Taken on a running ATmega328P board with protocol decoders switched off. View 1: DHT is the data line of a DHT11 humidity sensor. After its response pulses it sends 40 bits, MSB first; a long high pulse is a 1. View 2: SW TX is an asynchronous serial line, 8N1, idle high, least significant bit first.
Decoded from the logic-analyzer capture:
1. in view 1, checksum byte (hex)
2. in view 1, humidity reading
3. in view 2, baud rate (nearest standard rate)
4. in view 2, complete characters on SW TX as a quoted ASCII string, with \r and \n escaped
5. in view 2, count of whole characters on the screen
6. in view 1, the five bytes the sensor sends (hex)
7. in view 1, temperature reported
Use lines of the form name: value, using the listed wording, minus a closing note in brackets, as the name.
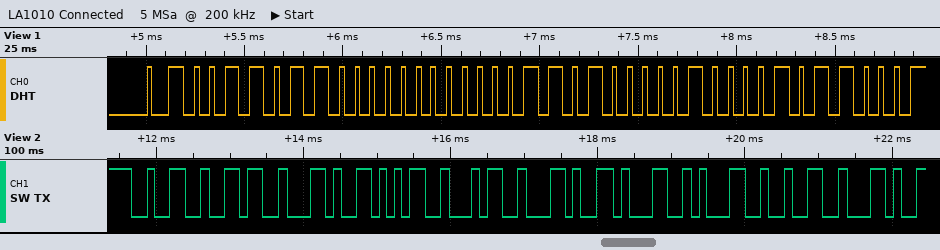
in view 1, checksum byte: 0x58
in view 1, humidity reading: 54 %
in view 2, baud rate: 9600 baud
in view 2, complete characters on SW TX as a quoted ASCII string, with \r and \n escaped: "26,54,112,"
in view 2, count of whole characters on the screen: 10
in view 1, the five bytes the sensor sends: 36 00 1A 08 58
in view 1, temperature reported: 26.8 °C
